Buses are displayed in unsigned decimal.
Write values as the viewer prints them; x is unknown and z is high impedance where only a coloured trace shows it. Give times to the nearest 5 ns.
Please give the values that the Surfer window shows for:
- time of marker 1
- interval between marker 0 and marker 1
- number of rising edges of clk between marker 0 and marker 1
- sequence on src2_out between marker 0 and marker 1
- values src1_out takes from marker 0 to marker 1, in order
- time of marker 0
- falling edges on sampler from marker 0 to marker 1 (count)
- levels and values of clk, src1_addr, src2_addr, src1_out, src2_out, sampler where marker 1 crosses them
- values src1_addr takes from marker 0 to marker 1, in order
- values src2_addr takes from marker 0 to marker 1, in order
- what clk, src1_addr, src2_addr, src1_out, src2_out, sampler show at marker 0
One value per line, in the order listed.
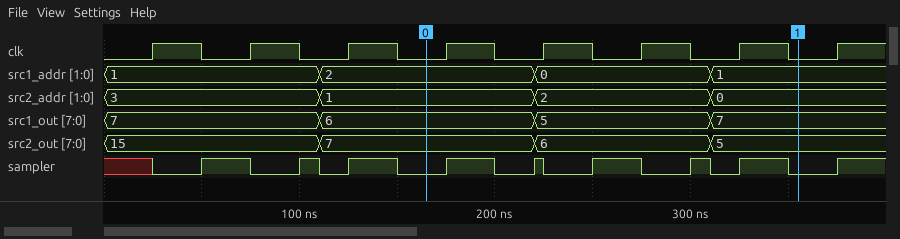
355 ns
190 ns
4
7, 6, 5
6, 5, 7
165 ns
5
clk=0, src1_addr=1, src2_addr=0, src1_out=7, src2_out=5, sampler=0
2, 0, 1
1, 2, 0
clk=0, src1_addr=2, src2_addr=1, src1_out=6, src2_out=7, sampler=0
